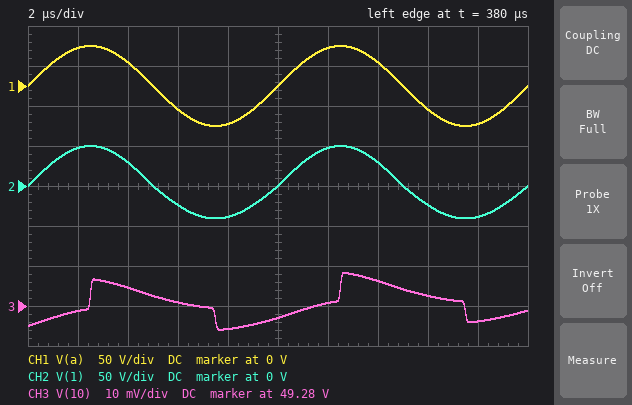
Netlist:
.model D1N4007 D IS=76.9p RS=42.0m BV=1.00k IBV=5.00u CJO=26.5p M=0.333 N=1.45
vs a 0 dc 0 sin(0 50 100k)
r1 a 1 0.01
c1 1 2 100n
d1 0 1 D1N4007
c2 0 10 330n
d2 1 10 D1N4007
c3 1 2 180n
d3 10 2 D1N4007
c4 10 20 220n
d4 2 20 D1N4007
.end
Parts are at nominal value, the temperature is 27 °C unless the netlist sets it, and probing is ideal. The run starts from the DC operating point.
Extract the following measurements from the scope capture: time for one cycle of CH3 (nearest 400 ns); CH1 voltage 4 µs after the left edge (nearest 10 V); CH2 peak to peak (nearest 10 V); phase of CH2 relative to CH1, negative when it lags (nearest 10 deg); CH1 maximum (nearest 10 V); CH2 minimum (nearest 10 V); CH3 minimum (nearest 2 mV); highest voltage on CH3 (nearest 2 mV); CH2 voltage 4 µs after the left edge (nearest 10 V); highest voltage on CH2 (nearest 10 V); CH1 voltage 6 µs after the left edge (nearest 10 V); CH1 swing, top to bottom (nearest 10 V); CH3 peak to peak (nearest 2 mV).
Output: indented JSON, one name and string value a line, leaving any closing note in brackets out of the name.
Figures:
{
  "time for one cycle of CH3": "10.0 µs",
  "CH1 voltage 4 µs after the left edge": "30 V",
  "CH2 peak to peak": "90 V",
  "phase of CH2 relative to CH1, negative when it lags": "0 deg",
  "CH1 maximum": "50 V",
  "CH2 minimum": "-40 V",
  "CH3 minimum": "49.274 V",
  "highest voltage on CH3": "49.288 V",
  "CH2 voltage 4 µs after the left edge": "30 V",
  "highest voltage on CH2": "50 V",
  "CH1 voltage 6 µs after the left edge": "-30 V",
  "CH1 swing, top to bottom": "100 V",
  "CH3 peak to peak": "14 mV"
}
